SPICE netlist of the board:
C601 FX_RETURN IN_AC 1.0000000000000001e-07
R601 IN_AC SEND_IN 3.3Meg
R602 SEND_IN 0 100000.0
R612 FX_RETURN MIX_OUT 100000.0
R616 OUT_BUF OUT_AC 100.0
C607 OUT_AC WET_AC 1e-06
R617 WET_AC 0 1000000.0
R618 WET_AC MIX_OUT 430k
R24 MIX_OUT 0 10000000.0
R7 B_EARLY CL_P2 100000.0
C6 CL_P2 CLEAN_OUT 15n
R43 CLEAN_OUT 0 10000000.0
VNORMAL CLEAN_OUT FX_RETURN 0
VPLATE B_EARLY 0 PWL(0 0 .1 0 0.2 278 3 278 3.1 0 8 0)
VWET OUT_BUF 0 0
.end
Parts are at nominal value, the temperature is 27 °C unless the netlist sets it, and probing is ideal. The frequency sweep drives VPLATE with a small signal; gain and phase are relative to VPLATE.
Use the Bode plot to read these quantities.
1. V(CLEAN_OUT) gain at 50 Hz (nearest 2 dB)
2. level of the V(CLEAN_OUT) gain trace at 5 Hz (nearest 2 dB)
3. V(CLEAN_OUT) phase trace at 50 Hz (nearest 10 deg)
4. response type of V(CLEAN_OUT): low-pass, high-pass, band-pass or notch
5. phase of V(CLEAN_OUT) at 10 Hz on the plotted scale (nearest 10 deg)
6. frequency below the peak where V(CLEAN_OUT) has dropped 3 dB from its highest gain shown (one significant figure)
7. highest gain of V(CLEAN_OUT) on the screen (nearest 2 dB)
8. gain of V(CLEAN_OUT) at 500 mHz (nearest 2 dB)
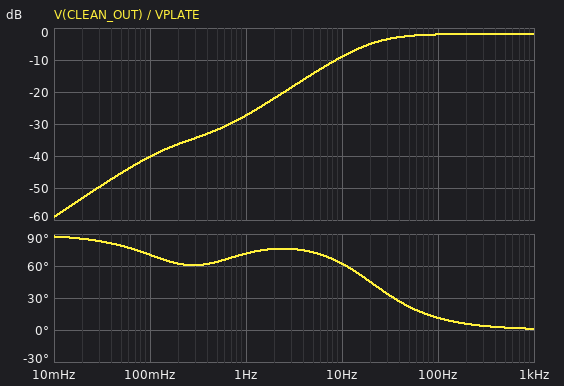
-2 dB
-14 dB
20 deg
high-pass
60 deg
20 Hz
-2 dB
-32 dB
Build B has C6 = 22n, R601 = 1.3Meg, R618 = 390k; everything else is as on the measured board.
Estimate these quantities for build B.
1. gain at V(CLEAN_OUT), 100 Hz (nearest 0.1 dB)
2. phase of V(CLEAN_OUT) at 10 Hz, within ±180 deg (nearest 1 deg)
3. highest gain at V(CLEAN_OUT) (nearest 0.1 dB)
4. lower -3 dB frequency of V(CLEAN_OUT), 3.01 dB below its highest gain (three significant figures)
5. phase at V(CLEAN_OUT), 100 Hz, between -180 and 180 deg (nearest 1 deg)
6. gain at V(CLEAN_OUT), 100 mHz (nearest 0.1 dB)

-2.3 dB
56 deg
-2.2 dB
16.7 Hz
9 deg
-37.0 dB
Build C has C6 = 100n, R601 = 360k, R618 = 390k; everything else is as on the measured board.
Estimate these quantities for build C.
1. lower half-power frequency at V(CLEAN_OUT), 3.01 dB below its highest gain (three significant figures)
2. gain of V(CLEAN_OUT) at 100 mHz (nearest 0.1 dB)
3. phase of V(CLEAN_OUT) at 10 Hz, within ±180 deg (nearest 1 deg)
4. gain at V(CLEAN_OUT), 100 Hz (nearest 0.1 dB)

4.95 Hz
-24.0 dB
21 deg
-3.2 dB
